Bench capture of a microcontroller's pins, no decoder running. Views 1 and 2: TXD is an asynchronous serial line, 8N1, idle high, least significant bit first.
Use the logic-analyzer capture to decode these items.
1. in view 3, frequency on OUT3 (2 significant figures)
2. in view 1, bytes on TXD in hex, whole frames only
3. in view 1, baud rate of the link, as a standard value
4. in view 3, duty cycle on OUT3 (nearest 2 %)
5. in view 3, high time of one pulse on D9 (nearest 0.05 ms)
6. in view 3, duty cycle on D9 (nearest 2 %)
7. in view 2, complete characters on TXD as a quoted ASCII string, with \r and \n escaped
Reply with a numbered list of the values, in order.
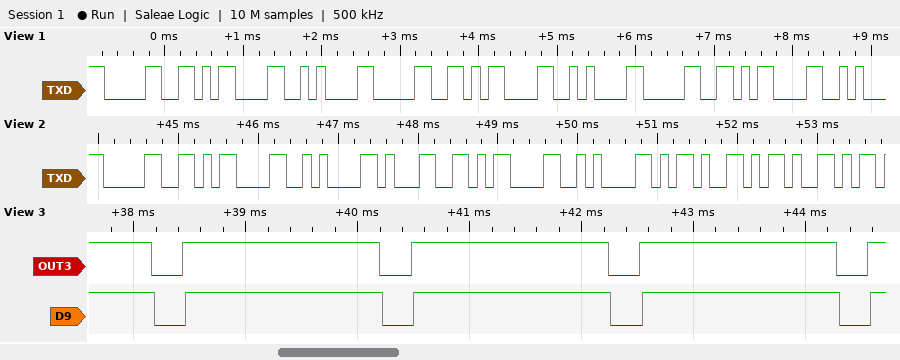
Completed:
1. 490 Hz
2. 0x30 0x0D 0x0A 0x30 0x0D 0x0A 0x30 0x0D
3. 9600 baud
4. 86 %
5. 1.75 ms
6. 86 %
7. "0\r\n1\r\n--"
